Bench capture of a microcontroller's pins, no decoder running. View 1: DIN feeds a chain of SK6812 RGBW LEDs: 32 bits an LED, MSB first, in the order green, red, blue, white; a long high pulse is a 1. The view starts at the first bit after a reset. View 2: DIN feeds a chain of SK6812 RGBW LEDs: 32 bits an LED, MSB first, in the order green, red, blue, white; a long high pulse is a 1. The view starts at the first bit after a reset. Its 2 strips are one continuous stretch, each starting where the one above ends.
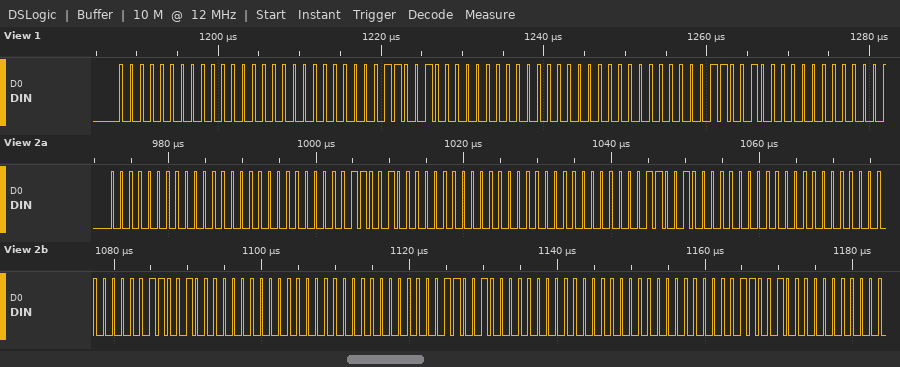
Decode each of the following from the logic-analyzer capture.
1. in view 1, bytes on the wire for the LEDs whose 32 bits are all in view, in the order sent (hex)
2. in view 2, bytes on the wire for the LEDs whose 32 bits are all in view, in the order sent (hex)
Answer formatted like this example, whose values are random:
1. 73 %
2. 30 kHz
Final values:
1. 00 00 00 32 00 00 00 32
2. 00 00 00 32 00 00 00 32 00 00 00 32 00 00 00 32 00 00 00 32
